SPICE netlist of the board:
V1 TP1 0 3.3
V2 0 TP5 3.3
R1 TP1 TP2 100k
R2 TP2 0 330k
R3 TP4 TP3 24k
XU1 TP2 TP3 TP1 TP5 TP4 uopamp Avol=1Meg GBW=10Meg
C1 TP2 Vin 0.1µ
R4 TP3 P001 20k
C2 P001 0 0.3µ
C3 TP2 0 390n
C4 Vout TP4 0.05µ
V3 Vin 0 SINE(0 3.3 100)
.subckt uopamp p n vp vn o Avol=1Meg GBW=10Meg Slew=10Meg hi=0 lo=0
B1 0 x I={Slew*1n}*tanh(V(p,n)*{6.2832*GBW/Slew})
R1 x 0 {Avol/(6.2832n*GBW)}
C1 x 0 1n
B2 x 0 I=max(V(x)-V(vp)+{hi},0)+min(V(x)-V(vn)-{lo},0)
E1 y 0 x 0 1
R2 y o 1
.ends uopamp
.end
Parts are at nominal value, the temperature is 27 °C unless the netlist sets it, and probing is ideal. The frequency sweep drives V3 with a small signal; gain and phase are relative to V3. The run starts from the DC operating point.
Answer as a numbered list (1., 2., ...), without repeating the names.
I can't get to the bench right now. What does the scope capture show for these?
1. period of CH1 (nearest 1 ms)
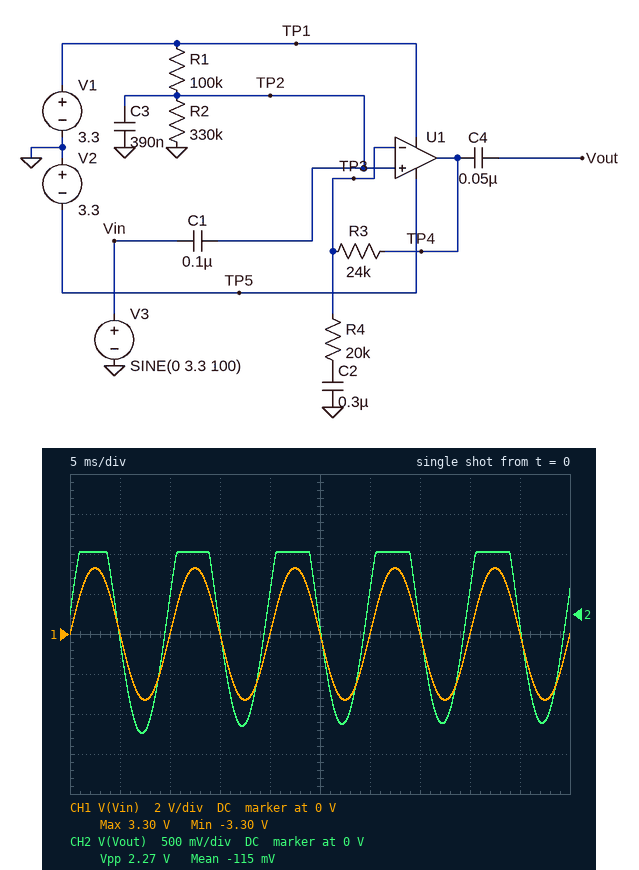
1. 10 ms
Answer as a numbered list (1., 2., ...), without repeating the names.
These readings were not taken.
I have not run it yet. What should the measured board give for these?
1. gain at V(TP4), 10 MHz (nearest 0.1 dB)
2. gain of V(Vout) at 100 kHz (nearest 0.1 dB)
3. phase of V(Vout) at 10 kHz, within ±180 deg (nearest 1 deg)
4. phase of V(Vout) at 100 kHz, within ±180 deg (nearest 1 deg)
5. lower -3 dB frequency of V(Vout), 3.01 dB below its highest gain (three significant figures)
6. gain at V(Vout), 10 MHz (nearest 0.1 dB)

1. -14.6 dB
2. -7.0 dB
3. 0 deg
4. -1 deg
5. 21.4 Hz
6. -14.6 dB
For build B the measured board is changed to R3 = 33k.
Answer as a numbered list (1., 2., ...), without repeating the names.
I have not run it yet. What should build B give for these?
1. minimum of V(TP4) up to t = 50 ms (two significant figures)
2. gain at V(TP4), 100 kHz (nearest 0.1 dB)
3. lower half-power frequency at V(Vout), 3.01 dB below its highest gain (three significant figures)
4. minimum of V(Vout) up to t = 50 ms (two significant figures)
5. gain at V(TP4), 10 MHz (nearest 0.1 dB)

1. 760 mV
2. -5.3 dB
3. 23.3 Hz
4. -1.8 V
5. -14.4 dB
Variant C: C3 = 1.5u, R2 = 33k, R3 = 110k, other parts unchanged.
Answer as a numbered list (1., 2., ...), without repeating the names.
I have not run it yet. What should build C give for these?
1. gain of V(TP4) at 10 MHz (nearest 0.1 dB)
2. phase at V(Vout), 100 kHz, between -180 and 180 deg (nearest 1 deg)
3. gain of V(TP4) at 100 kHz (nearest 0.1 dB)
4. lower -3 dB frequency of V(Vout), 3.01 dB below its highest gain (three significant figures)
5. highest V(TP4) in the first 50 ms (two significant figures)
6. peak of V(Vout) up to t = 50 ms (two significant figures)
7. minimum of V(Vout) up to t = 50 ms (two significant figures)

1. -24.2 dB
2. -4 deg
3. -7.8 dB
4. 26.5 Hz
5. 2.1 V
6. 1.3 V
7. -1.4 V
